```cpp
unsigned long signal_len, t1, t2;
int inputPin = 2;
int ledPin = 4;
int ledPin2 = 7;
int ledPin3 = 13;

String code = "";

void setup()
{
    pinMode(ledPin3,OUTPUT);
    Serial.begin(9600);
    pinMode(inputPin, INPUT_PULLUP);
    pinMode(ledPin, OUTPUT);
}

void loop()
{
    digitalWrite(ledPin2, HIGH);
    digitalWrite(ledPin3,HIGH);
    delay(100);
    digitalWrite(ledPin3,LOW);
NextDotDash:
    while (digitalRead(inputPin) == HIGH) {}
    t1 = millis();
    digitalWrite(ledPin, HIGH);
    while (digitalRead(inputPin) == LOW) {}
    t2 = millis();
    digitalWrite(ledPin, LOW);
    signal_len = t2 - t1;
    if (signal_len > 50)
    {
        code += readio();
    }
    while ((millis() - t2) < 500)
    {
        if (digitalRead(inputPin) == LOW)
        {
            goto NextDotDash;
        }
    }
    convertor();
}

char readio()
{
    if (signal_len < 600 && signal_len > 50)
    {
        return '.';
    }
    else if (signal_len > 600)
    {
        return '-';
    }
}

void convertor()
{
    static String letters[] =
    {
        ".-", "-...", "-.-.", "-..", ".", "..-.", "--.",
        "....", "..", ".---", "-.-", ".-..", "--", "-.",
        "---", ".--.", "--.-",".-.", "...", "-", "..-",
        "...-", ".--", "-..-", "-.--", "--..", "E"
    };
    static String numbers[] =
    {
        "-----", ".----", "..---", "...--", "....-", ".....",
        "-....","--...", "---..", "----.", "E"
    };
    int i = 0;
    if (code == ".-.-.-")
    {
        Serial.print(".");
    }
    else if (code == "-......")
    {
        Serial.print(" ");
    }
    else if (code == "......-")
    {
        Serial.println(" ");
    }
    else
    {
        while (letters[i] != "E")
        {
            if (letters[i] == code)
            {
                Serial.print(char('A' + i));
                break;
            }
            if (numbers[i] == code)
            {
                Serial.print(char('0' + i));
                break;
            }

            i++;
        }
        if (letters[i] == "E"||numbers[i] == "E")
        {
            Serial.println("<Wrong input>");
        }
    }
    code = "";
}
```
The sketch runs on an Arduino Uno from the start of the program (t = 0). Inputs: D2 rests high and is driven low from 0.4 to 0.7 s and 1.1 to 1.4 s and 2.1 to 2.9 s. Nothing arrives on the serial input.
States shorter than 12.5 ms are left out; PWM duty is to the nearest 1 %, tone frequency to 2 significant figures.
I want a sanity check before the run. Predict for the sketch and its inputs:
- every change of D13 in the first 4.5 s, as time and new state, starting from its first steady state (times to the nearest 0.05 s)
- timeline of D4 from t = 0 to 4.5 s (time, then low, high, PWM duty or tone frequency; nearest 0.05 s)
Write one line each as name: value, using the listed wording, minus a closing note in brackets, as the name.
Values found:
every change of D13 in the first 4.5 s, as time and new state, starting from its first steady state: 0 s high; 0.1 s low; 1.9 s high; 2 s low; 3.4 s high; 3.5 s low
timeline of D4 from t = 0 to 4.5 s: 0 s low; 0.4 s high; 0.7 s low; 1.1 s high; 1.4 s low; 2.1 s high; 2.9 s low
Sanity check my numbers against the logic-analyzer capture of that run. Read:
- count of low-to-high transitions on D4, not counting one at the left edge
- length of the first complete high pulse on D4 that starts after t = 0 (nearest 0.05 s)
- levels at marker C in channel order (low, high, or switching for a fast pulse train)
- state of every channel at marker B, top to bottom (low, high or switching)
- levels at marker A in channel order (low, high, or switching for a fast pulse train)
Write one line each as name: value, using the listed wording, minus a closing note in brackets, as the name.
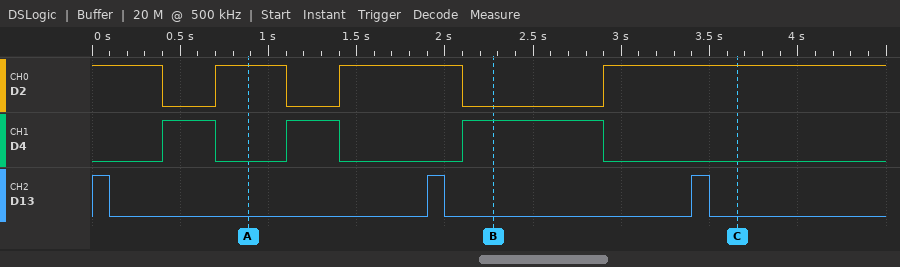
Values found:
count of low-to-high transitions on D4, not counting one at the left edge: 3
length of the first complete high pulse on D4 that starts after t = 0: 0.30 s
levels at marker C in channel order: D2 high, D4 low, D13 low
state of every channel at marker B, top to bottom: D2 low, D4 high, D13 low
levels at marker A in channel order: D2 high, D4 low, D13 low
